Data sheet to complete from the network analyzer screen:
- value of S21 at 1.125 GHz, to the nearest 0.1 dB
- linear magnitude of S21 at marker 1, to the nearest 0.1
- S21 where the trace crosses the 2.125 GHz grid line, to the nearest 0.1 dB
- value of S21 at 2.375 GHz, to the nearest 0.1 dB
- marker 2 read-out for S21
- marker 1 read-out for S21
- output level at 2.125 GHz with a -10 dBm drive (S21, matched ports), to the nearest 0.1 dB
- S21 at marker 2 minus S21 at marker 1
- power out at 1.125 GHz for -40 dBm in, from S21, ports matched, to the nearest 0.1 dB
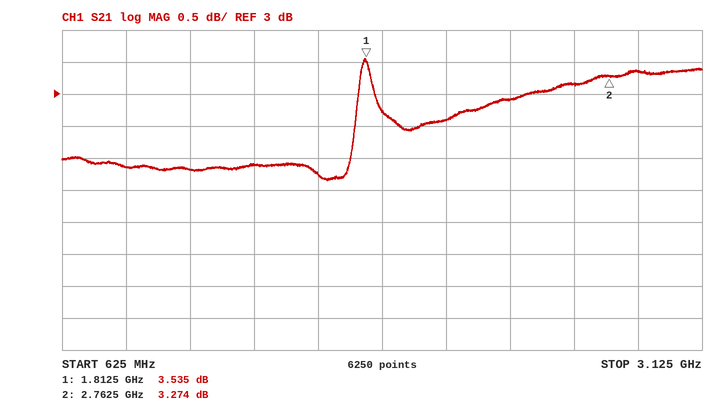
1.8 dB
1.5
2.6 dB
2.9 dB
3.274 dB
3.535 dB
-7.4 dBm
-0.261 dB
-38.2 dBm
